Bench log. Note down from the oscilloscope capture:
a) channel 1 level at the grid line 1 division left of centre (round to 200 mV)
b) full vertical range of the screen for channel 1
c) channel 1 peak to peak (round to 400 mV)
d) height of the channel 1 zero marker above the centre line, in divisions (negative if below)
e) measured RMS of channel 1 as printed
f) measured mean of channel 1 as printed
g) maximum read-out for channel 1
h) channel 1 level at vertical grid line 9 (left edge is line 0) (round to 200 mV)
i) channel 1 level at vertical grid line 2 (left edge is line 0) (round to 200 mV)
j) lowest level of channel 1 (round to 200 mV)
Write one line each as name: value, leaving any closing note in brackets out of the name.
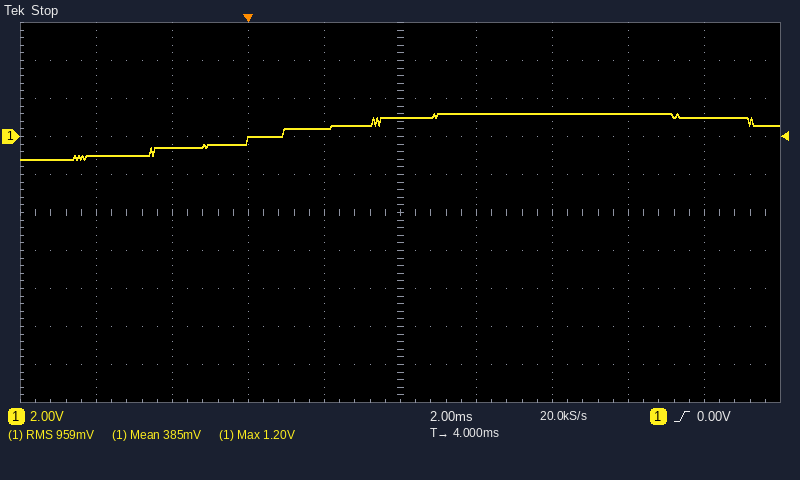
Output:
channel 1 level at the grid line 1 division left of centre: 400 mV
full vertical range of the screen for channel 1: 20 V
channel 1 peak to peak: 2.4 V
height of the channel 1 zero marker above the centre line, in divisions: +2.0 div
measured RMS of channel 1 as printed: 959 mV
measured mean of channel 1 as printed: 385 mV
maximum read-out for channel 1: 1.20 V
channel 1 level at vertical grid line 9 (left edge is line 0): 1.0 V
channel 1 level at vertical grid line 2 (left edge is line 0): -600 mV
lowest level of channel 1: -1.2 V
